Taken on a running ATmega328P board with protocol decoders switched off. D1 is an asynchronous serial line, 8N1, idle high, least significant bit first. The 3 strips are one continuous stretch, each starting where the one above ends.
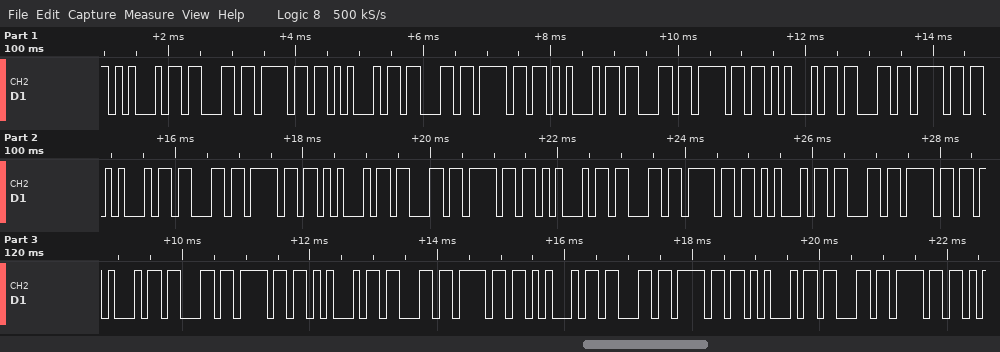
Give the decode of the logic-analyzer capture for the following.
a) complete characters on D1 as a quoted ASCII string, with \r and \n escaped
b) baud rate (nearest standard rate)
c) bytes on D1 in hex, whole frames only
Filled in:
"EcoEcoEcoEcoEcoEcoEcoEcoEcoEcoEcoEco"
9600 baud
45 63 6F 45 63 6F 45 63 6F 45 63 6F 45 63 6F 45 63 6F 45 63 6F 45 63 6F 45 63 6F 45 63 6F 45 63 6F 45 63 6F
